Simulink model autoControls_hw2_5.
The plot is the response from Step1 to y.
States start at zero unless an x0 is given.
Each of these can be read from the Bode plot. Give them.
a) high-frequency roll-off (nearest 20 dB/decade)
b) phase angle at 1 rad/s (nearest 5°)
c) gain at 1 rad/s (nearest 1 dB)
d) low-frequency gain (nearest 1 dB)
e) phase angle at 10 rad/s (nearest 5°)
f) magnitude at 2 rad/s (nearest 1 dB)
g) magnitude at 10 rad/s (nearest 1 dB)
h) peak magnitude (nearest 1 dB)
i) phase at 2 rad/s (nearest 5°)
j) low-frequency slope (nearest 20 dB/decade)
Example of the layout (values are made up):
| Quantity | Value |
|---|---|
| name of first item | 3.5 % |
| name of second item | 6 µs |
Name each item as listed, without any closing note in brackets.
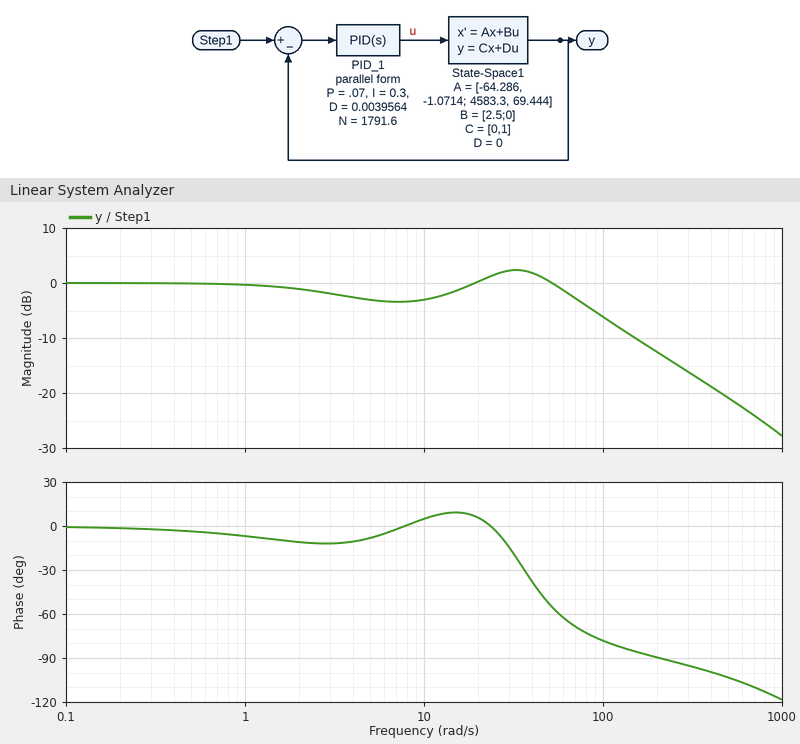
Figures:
| Quantity | Value |
|---|---|
| high-frequency roll-off | -20 dB/decade |
| phase angle at 1 rad/s | -5° |
| gain at 1 rad/s | 0 dB |
| low-frequency gain | 0 dB |
| phase angle at 10 rad/s | 5° |
| magnitude at 2 rad/s | -1 dB |
| magnitude at 10 rad/s | -3 dB |
| peak magnitude | 2 dB |
| phase at 2 rad/s | -10° |
| low-frequency slope | 0 dB/decade |
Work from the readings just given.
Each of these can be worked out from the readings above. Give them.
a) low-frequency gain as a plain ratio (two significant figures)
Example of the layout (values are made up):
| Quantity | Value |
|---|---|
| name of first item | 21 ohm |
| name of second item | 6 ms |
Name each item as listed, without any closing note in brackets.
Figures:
| Quantity | Value |
|---|---|
| low-frequency gain as a plain ratio | 1.0 |
